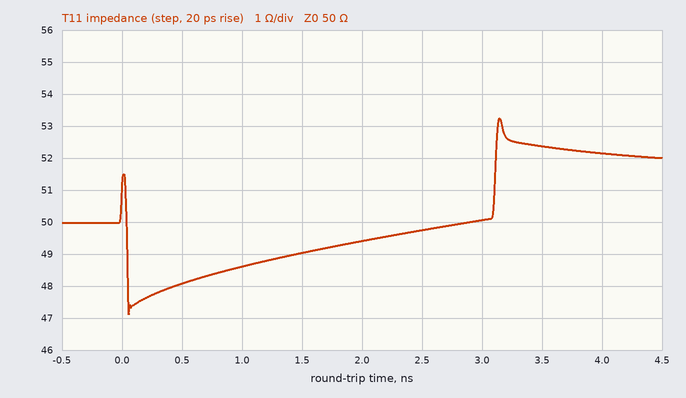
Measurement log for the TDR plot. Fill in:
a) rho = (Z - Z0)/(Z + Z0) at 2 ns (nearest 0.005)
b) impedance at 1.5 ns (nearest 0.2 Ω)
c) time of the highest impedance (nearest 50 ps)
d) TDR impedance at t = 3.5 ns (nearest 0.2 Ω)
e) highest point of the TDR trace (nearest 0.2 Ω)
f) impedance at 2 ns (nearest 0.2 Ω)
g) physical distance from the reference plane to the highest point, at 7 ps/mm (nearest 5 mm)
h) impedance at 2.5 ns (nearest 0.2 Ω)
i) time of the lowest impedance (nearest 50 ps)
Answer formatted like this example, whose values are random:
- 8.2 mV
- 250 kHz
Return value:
- -0.005
- 49.0 Ω
- 3.15 ns
- 52.4 Ω
- 53.2 Ω
- 49.4 Ω
- 225 mm
- 49.8 Ω
- 50 ps
